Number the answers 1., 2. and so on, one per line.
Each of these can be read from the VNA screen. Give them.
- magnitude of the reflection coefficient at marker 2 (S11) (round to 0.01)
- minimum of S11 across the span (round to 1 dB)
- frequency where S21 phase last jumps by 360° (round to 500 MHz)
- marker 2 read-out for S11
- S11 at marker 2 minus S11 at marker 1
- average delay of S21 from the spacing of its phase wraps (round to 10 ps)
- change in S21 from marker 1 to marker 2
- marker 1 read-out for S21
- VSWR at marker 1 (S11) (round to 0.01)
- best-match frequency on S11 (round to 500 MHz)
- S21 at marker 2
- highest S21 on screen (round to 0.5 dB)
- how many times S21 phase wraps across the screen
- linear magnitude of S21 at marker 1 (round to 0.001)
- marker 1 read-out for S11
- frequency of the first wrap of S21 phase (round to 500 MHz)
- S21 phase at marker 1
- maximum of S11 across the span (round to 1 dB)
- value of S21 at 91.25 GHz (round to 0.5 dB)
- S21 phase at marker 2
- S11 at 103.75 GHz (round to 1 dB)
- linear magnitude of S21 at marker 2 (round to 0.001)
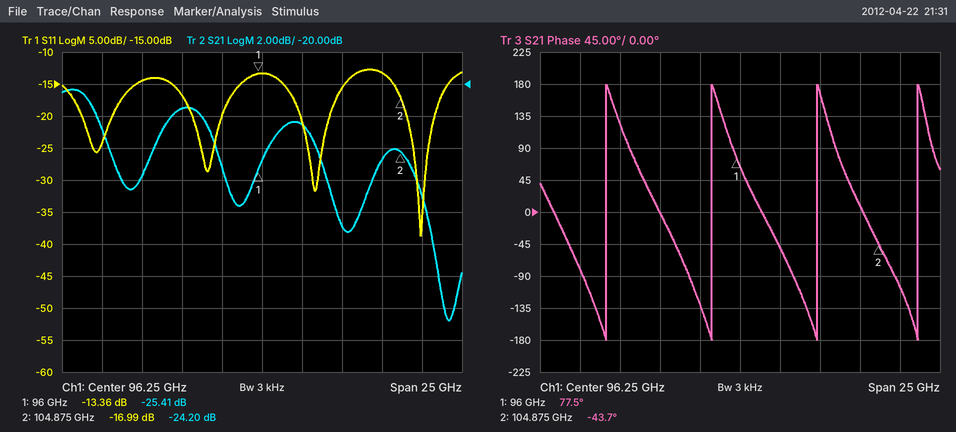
1. 0.14
2. -39 dB
3. 107.5 GHz
4. -16.99 dB
5. -3.63 dB
6. 150 ps
7. 1.21 dB
8. -25.41 dB
9. 1.55
10. 106.0 GHz
11. -24.20 dB
12. -20.5 dB
13. 4
14. 0.054
15. -13.36 dB
16. 88.0 GHz
17. 77.5°
18. -13 dB
19. -21.5 dB
20. -43.7°
21. -13 dB
22. 0.062
